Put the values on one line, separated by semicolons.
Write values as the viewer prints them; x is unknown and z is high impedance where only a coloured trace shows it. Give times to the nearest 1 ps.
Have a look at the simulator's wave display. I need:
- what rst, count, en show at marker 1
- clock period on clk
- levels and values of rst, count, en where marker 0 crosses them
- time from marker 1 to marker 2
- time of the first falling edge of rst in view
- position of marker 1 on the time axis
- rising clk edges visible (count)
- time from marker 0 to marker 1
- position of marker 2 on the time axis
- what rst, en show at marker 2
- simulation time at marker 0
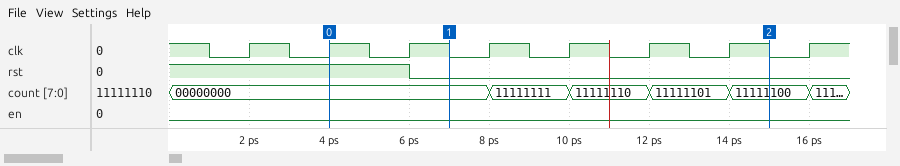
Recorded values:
rst=0, count=00000000, en=0; 2 ps; rst=1, count=00000000, en=0; 8 ps; 6 ps; 7 ps; 8; 3 ps; 15 ps; rst=0, en=0; 4 ps
